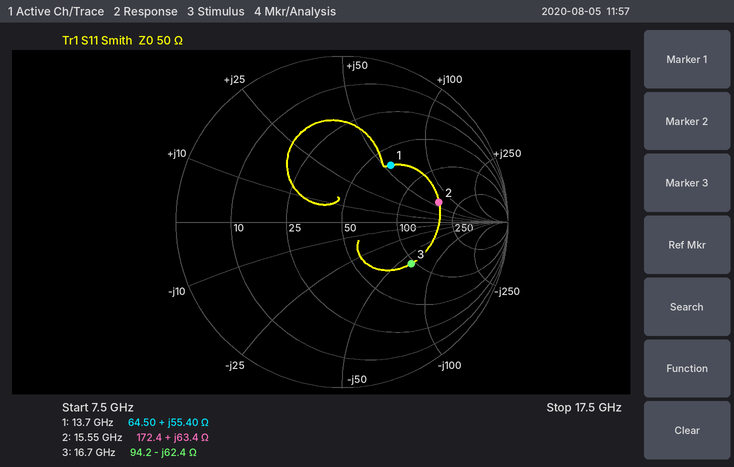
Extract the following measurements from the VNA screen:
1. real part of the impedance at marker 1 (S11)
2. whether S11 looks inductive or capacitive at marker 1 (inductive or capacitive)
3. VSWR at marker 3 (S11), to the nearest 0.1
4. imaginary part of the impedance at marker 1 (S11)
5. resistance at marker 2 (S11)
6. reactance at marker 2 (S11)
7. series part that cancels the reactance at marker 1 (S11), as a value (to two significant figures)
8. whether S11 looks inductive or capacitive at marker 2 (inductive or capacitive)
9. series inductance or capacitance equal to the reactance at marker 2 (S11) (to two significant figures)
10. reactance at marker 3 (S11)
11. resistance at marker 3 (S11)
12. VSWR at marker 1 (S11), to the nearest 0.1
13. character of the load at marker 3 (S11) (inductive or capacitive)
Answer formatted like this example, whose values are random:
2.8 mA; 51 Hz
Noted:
64.50 Ω; inductive; 2.9; +55.40 Ω; 172.4 Ω; +63.4 Ω; 210 fF; inductive; 650 pH; -62.4 Ω; 94.2 Ω; 2.6; capacitive
